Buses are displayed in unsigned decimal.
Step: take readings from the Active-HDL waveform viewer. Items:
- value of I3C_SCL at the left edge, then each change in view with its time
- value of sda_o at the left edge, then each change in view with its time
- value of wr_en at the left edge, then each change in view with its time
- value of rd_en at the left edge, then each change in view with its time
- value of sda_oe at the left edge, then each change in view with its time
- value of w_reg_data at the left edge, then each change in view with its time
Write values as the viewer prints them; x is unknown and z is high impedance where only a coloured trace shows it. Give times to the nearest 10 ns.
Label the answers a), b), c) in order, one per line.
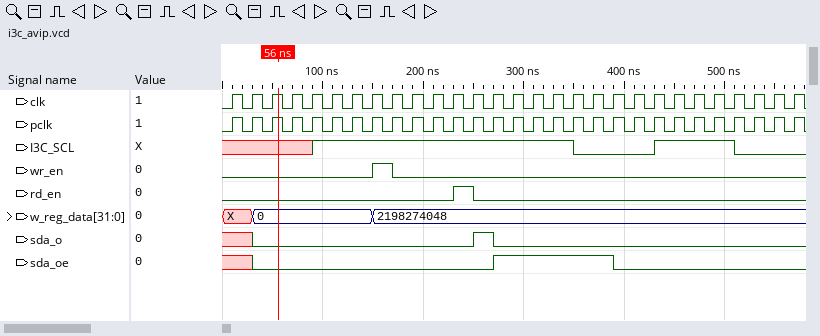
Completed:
a) x, 1 at 90 ns, 0 at 350 ns, 1 at 430 ns, 0 at 510 ns
b) x, 0 at 30 ns, 1 at 250 ns, 0 at 270 ns
c) 0, 1 at 150 ns, 0 at 170 ns
d) 0, 1 at 230 ns, 0 at 250 ns
e) x, 0 at 30 ns, 1 at 270 ns, 0 at 390 ns
f) X, 0 at 30 ns, 2198274048 at 150 ns
